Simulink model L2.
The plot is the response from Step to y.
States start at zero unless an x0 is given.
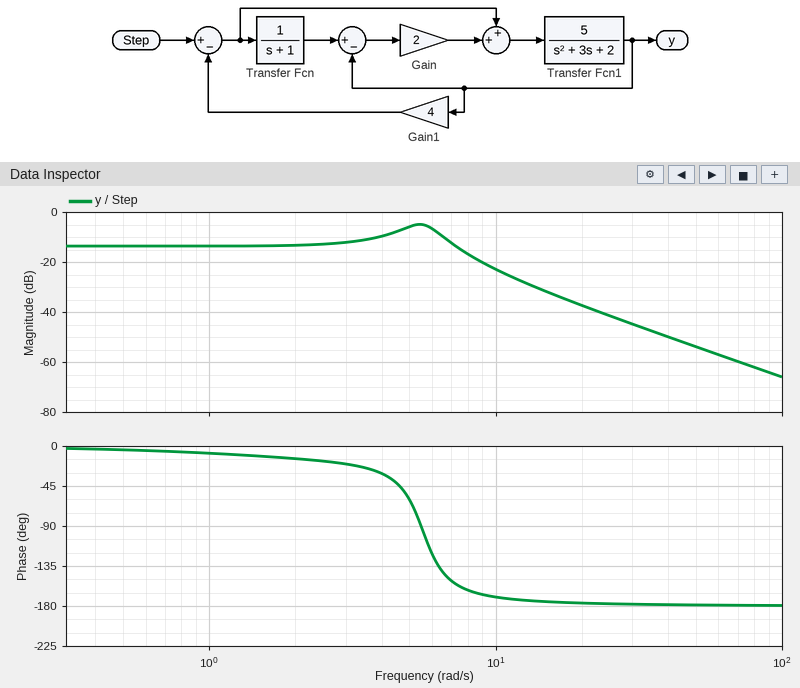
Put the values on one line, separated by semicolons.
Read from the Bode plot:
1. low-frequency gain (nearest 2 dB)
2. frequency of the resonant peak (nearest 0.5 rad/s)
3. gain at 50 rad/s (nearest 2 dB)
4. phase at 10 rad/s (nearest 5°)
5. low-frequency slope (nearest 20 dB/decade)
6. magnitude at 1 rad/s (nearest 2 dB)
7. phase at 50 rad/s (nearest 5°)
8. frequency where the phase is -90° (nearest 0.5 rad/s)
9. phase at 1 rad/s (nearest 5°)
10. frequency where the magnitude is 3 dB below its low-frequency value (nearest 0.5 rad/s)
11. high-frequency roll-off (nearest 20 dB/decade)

-14 dB; 5.5 rad/s; -54 dB; -170°; 0 dB/decade; -14 dB; -180°; 5.5 rad/s; -10°; 8.0 rad/s; -40 dB/decade
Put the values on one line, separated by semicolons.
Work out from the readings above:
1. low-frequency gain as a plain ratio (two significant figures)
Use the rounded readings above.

0.20
